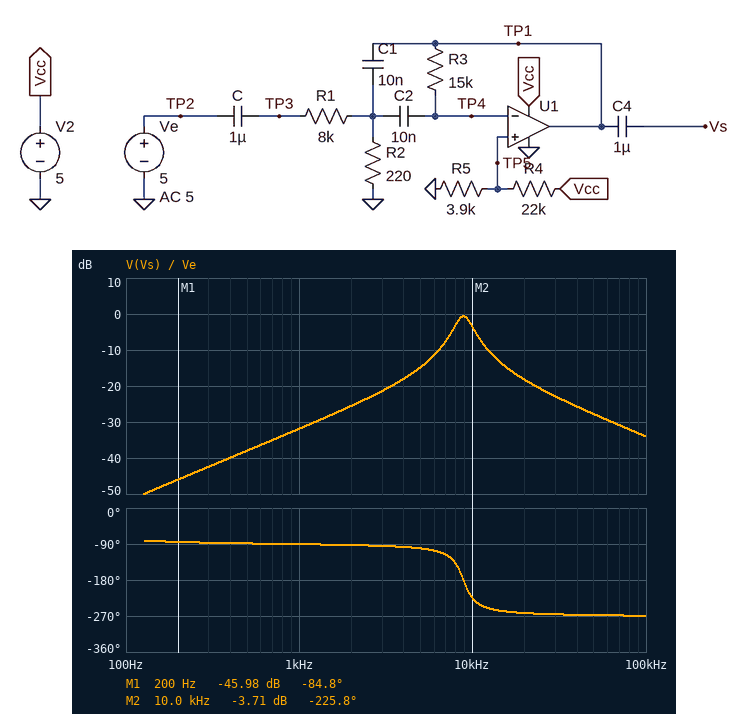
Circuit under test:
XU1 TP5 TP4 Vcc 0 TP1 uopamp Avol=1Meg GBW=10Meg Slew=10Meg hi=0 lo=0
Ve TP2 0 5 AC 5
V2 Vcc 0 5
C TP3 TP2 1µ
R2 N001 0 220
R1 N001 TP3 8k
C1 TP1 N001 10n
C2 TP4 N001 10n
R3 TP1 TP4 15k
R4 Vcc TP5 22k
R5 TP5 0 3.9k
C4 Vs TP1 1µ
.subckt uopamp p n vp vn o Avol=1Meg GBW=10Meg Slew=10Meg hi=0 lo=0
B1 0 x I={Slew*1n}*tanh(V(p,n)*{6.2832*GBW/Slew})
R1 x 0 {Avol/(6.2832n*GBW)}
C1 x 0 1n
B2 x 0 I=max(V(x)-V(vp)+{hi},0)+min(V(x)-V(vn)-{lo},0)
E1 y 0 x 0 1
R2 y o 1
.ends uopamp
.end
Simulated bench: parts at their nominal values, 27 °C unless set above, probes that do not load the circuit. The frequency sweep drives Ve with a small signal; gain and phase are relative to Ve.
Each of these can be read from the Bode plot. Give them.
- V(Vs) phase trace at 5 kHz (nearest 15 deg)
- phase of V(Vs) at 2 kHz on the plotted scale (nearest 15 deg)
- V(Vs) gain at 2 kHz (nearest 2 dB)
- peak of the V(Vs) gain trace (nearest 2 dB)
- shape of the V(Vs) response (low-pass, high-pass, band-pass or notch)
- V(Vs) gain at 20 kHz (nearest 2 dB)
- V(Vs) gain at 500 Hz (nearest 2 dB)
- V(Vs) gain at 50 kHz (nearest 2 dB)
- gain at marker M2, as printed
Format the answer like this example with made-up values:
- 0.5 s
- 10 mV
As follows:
- -105 deg
- -90 deg
- -26 dB
- 0 dB
- band-pass
- -18 dB
- -38 dB
- -28 dB
- -3.71 dB
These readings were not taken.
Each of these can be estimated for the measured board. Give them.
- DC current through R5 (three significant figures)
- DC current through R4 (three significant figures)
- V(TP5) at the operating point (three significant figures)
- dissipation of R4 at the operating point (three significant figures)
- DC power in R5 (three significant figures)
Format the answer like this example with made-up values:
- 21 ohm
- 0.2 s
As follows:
- 193 µA
- 193 µA
- 753 mV
- 820 µW
- 145 µW
